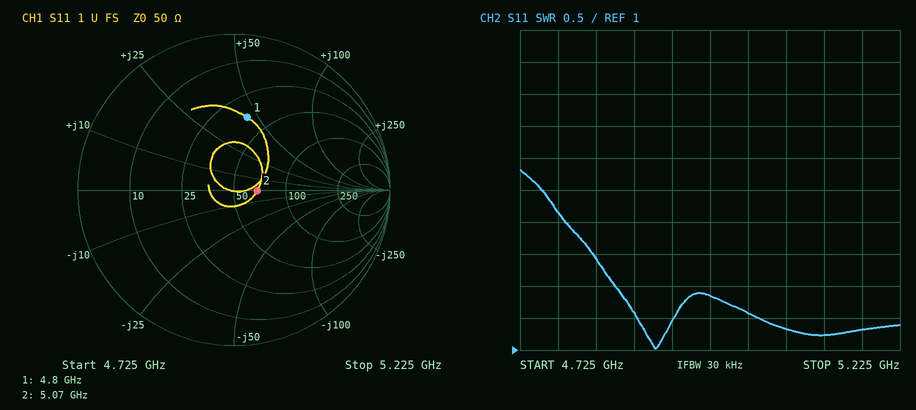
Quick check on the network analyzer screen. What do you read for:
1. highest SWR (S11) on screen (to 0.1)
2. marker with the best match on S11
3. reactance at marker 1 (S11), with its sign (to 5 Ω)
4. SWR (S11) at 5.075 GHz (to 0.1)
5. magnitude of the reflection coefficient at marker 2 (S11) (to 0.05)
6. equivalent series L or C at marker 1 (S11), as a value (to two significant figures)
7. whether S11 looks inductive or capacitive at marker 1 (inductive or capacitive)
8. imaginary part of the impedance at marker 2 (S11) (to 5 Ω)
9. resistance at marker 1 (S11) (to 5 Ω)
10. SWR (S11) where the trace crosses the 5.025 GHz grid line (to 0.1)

3.8
marker 2
+45 Ω
1.3
0.15
1.5 nH
inductive
0 Ω
35 Ω
1.6
